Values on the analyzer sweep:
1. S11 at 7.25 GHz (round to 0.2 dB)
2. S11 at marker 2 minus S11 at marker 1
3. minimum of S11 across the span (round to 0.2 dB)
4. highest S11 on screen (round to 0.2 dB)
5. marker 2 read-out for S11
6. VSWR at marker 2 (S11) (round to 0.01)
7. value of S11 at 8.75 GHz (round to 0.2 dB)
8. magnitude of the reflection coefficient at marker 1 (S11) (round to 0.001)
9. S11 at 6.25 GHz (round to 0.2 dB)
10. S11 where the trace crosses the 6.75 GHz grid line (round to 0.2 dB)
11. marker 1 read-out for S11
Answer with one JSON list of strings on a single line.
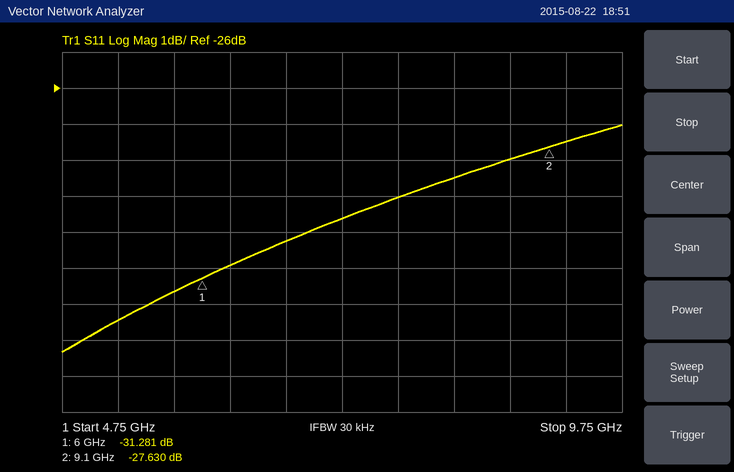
["-29.6 dB", "3.651 dB", "-33.4 dB", "-27.0 dB", "-27.630 dB", "1.09", "-28.0 dB", "0.027", "-31.0 dB", "-30.2 dB", "-31.281 dB"]
